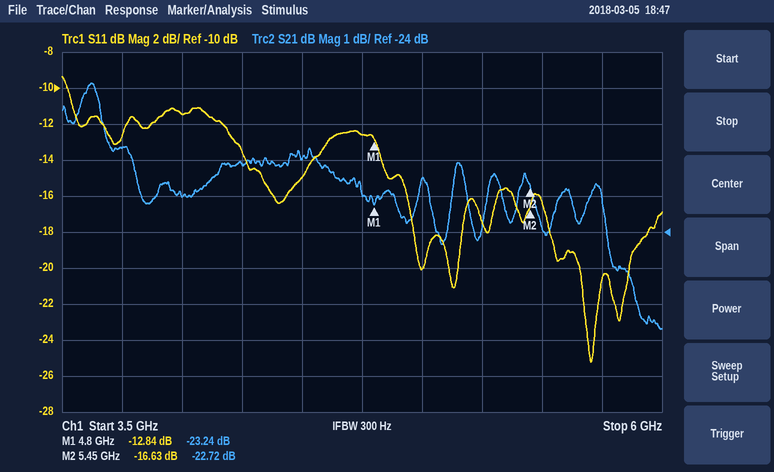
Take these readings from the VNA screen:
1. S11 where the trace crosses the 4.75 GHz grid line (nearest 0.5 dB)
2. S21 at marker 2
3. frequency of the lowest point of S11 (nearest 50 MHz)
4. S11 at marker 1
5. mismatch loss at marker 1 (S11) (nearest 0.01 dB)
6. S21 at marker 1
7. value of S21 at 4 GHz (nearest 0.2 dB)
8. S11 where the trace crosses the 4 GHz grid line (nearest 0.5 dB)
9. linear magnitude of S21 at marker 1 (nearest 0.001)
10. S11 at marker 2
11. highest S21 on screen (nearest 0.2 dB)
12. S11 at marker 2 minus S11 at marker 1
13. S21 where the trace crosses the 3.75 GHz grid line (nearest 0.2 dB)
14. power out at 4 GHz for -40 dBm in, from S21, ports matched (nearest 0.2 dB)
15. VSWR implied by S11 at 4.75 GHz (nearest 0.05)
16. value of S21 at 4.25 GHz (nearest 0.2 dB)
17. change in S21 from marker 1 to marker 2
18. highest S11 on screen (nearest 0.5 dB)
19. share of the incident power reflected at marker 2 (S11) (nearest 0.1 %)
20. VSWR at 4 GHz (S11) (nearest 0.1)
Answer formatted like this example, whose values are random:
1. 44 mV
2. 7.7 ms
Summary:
1. -12.5 dB
2. -22.72 dB
3. 5.70 GHz
4. -12.84 dB
5. 0.23 dB
6. -23.24 dB
7. -23.0 dB
8. -11.5 dB
9. 0.069
10. -16.63 dB
11. -19.8 dB
12. -3.79 dB
13. -21.6 dB
14. -63.0 dBm
15. 1.60
16. -22.2 dB
17. 0.52 dB
18. -9.5 dB
19. 2.2 %
20. 1.7
